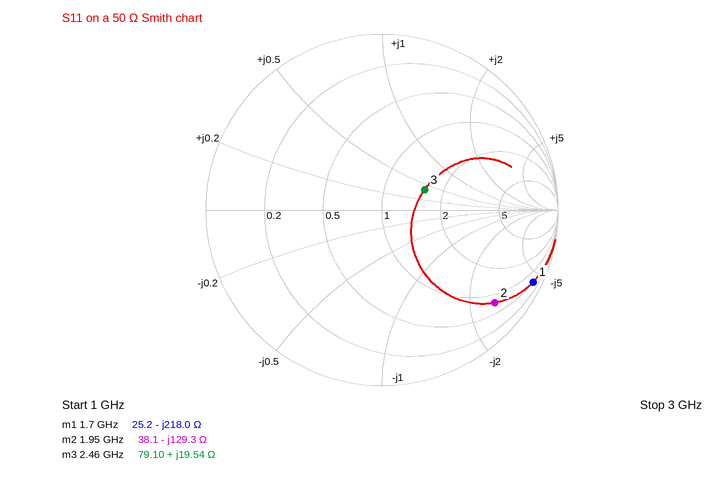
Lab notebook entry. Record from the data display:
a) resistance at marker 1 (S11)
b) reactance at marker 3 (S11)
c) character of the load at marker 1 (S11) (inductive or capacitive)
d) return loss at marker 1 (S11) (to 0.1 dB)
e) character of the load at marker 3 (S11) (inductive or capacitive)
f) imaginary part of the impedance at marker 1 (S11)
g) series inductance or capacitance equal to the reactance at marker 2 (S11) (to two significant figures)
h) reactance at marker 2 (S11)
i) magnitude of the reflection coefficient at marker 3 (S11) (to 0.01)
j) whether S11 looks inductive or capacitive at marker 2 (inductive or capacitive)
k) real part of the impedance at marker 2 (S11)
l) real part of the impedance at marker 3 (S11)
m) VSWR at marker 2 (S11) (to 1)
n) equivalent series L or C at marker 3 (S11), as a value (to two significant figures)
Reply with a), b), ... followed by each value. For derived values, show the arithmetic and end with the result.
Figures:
a) 25.2 Ω
b) +19.54 Ω
c) capacitive
d) 0.4 dB
e) inductive
f) -218.0 Ω
g) C = 1/(2π × 1.95 GHz × 129.3 Ω) ≈ 631 fF, so 630 fF to two significant figures
h) -129.3 Ω
i) 0.27
j) capacitive
k) 38.1 Ω
l) 79.10 Ω
m) 11
n) L = 19.54 Ω/(2π × 2.46 GHz) ≈ 1.3 nH
